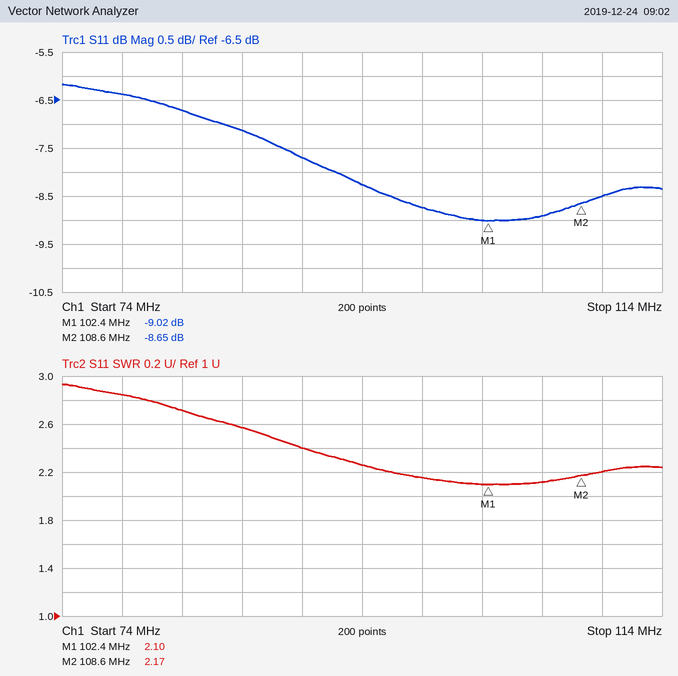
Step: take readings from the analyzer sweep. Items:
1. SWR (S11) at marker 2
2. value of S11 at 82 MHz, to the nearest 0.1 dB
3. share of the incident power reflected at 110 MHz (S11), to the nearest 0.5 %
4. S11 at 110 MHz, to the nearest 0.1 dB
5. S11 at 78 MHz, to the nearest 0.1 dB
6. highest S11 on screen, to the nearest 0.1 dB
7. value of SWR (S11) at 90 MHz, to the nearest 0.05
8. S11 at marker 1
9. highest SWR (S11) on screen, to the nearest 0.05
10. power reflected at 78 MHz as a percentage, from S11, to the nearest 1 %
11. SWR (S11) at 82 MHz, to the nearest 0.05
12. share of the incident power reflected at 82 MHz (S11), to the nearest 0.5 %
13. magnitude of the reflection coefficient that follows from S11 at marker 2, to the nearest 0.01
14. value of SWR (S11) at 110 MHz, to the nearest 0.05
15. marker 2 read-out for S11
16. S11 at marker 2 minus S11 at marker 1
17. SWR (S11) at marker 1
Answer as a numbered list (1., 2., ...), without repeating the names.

1. 2.17
2. -6.7 dB
3. 14.0 %
4. -8.5 dB
5. -6.4 dB
6. -6.2 dB
7. 2.40
8. -9.02 dB
9. 2.95
10. 23 %
11. 2.70
12. 21.5 %
13. 0.37
14. 2.20
15. -8.65 dB
16. 0.37 dB
17. 2.10
